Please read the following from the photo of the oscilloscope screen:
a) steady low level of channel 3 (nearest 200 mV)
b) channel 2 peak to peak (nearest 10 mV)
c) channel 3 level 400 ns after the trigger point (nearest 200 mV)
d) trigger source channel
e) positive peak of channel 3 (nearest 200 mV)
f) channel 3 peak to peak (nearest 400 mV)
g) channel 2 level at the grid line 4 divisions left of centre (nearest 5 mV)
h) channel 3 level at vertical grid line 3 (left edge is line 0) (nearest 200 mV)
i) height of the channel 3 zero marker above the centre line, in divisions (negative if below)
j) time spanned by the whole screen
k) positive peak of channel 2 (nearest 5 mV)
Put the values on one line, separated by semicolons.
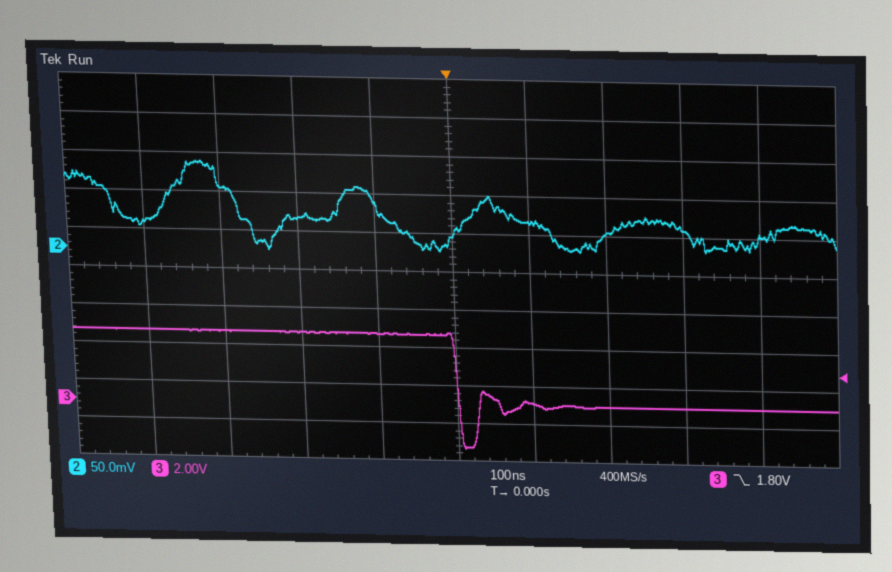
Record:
0.0 V; 110 mV; 0.0 V; channel 3; 3.8 V; 6.0 V; 35 mV; 3.8 V; -3.5 div; 1 µs; 115 mV
